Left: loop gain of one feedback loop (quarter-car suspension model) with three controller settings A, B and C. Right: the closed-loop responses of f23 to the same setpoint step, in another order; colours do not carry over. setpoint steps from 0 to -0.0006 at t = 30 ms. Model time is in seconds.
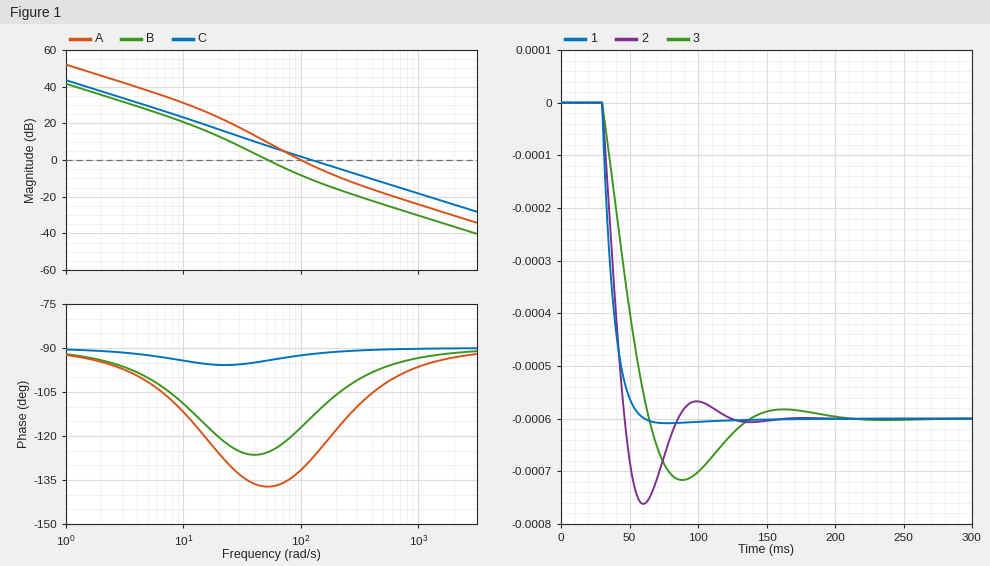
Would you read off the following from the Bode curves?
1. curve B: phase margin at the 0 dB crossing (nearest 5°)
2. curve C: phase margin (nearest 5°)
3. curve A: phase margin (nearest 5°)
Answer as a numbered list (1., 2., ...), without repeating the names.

1. 55°
2. 90°
3. 50°
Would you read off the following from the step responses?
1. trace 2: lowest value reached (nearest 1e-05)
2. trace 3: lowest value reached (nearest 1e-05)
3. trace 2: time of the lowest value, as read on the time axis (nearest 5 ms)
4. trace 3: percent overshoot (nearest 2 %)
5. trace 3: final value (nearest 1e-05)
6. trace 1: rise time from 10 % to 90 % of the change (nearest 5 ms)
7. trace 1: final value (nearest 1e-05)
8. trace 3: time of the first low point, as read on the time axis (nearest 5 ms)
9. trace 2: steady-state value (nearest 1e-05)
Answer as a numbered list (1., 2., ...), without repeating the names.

1. -0.00076
2. -0.00072
3. 60 ms
4. 20 %
5. -0.00060
6. 15 ms
7. -0.00060
8. 90 ms
9. -0.00060
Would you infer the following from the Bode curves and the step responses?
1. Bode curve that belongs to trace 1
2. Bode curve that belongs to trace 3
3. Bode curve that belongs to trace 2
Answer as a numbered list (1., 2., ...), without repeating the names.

1. C
2. B
3. A
